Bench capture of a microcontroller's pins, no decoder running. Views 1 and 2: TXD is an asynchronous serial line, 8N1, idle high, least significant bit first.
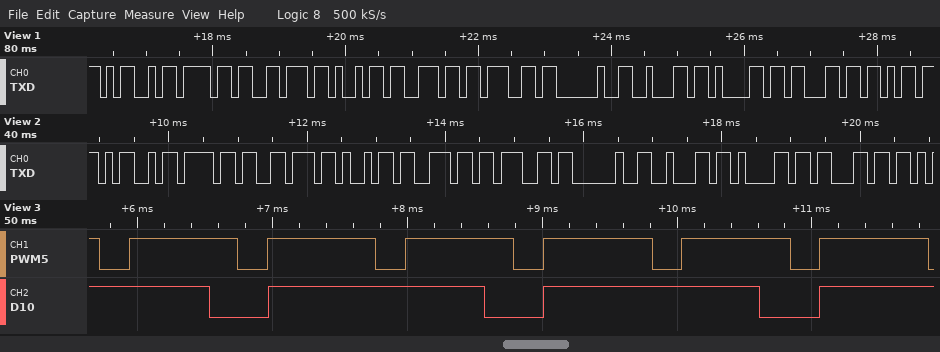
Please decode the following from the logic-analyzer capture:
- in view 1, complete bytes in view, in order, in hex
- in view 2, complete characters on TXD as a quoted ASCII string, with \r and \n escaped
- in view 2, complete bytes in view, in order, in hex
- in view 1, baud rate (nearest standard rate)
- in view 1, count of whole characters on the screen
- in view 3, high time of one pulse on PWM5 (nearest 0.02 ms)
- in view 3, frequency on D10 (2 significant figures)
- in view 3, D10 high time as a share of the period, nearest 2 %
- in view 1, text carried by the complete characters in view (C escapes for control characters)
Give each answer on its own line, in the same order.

0x4D 0x6F 0x76 0x69 0x6E 0x67 0x20 0x62 0x61 0x63 0x6B
"Moving bac"
0x4D 0x6F 0x76 0x69 0x6E 0x67 0x20 0x62 0x61 0x63
9600 baud
11
0.80 ms
490 Hz
78 %
"Moving back"
